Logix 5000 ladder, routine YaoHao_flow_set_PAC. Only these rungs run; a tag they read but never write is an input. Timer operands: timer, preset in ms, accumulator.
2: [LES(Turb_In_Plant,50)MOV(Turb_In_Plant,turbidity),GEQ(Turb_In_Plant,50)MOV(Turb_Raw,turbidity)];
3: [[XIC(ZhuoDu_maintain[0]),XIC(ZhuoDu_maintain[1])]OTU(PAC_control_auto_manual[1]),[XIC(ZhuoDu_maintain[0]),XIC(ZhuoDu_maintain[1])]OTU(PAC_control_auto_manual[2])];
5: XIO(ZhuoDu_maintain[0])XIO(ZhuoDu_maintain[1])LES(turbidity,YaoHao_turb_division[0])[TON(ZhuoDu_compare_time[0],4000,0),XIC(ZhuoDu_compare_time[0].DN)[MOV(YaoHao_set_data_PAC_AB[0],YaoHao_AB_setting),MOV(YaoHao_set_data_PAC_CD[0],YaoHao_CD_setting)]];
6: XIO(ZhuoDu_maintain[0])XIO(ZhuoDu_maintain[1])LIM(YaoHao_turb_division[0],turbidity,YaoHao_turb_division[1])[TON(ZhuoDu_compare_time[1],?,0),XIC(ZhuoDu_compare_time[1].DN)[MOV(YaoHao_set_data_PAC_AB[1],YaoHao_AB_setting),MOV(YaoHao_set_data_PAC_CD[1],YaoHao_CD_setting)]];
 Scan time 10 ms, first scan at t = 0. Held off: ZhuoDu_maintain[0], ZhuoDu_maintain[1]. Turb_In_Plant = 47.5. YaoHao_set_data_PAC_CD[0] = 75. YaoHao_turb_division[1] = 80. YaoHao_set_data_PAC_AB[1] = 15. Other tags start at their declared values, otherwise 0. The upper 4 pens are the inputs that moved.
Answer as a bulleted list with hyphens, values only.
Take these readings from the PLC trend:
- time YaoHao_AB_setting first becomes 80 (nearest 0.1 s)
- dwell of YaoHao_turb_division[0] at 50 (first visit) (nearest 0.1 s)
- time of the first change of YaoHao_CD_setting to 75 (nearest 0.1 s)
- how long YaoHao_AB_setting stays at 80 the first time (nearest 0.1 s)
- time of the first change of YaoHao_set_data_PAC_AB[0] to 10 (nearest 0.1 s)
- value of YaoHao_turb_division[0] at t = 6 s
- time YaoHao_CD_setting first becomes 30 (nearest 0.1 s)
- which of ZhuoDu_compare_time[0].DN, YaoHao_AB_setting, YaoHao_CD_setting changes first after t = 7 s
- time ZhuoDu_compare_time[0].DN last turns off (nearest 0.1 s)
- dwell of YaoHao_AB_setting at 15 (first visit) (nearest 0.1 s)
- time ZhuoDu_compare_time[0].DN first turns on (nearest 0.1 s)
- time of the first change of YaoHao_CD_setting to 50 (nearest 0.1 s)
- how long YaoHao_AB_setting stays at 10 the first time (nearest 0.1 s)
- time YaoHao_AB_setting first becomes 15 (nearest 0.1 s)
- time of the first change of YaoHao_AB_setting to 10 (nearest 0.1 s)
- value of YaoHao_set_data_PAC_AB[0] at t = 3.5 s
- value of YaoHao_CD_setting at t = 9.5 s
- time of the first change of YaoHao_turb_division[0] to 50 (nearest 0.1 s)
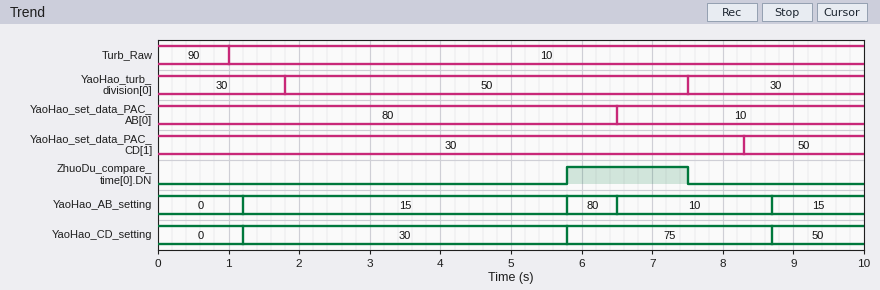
- 5.8 s
- 5.7 s
- 5.8 s
- 0.7 s
- 6.5 s
- 50
- 1.2 s
- ZhuoDu_compare_time[0].DN
- 7.5 s
- 4.6 s
- 5.8 s
- 8.7 s
- 2.2 s
- 1.2 s
- 6.5 s
- 80
- 50
- 1.8 s
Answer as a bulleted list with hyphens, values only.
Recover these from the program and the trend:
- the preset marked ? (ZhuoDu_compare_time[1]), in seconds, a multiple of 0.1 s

- 1.2 s
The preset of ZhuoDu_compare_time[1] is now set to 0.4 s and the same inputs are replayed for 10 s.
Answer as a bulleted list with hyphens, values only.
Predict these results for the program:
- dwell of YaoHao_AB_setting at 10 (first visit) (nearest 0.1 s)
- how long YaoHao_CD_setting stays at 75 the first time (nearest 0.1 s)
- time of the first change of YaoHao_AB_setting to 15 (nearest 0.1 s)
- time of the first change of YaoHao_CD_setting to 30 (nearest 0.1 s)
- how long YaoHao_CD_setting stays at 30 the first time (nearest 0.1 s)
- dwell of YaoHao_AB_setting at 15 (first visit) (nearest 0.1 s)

- 1.4 s
- 2.1 s
- 0.4 s
- 0.4 s
- 5.4 s
- 5.4 s
